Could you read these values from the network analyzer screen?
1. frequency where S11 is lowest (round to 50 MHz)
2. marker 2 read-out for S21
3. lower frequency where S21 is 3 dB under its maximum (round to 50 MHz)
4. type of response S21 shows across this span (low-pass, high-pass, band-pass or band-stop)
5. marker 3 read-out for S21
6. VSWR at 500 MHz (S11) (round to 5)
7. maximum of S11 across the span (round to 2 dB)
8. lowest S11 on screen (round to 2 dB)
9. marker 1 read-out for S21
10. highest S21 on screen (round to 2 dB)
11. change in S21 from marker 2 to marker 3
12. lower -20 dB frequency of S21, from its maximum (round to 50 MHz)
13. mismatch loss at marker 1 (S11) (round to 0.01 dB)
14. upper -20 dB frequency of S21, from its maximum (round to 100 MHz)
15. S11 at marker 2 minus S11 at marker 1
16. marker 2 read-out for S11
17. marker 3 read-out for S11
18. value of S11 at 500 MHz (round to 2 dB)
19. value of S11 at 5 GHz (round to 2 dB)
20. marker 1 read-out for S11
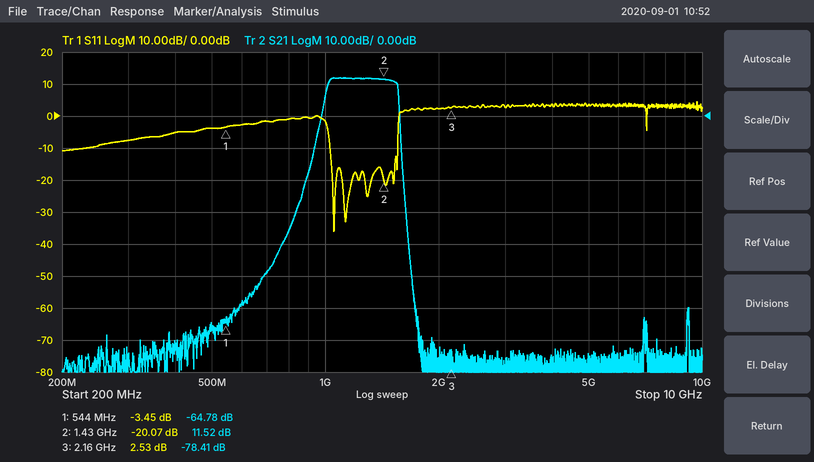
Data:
1.05 GHz
11.52 dB
1.00 GHz
band-pass
-78.41 dB
5
4 dB
-36 dB
-64.78 dB
12 dB
-89.93 dB
950 MHz
2.61 dB
1.6 GHz
-16.62 dB
-20.07 dB
2.53 dB
-4 dB
4 dB
-3.45 dB
